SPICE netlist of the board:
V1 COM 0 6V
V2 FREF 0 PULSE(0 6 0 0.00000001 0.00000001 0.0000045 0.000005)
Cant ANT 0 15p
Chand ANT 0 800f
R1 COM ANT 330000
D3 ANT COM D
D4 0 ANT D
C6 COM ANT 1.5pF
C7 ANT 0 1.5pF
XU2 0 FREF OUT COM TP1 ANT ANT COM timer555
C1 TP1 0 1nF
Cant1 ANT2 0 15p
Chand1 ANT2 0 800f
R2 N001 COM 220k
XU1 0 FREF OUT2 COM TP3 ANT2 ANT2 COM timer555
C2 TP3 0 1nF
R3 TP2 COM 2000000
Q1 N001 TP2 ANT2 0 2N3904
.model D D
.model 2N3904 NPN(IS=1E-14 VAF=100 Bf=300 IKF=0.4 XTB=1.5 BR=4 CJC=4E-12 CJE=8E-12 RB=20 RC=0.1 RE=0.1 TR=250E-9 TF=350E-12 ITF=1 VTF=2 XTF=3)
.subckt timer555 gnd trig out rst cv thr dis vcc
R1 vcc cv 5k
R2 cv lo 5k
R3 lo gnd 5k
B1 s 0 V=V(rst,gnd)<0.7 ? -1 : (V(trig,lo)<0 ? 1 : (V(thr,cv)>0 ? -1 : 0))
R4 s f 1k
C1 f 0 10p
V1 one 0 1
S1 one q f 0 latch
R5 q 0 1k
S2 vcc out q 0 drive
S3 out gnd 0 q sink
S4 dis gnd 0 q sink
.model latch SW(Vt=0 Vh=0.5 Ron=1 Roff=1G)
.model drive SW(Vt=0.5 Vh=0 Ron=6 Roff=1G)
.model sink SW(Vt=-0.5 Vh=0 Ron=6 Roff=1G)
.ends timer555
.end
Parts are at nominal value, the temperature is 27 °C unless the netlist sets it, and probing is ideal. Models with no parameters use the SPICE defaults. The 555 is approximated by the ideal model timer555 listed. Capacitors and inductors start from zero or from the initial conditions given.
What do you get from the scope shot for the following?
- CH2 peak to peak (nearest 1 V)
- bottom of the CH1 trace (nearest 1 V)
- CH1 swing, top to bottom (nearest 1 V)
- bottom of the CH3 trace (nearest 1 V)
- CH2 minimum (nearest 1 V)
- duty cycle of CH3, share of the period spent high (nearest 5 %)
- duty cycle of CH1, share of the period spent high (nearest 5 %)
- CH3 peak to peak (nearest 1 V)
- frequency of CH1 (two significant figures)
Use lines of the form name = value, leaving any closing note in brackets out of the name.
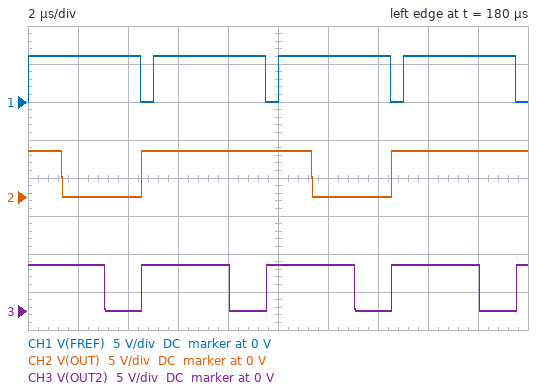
CH2 peak to peak = 6 V
bottom of the CH1 trace = 0 V
CH1 swing, top to bottom = 6 V
bottom of the CH3 trace = 0 V
CH2 minimum = 0 V
duty cycle of CH3, share of the period spent high = 70 %
duty cycle of CH1, share of the period spent high = 90 %
CH3 peak to peak = 6 V
frequency of CH1 = 200 kHz
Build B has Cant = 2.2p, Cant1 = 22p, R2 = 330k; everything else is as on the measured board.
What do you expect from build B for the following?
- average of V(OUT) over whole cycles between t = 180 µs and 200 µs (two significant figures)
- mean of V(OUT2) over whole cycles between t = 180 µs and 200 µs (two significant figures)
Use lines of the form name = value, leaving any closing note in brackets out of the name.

average of V(OUT) over whole cycles between t = 180 µs and 200 µs = 2.6 V
mean of V(OUT2) over whole cycles between t = 180 µs and 200 µs = 4.4 V
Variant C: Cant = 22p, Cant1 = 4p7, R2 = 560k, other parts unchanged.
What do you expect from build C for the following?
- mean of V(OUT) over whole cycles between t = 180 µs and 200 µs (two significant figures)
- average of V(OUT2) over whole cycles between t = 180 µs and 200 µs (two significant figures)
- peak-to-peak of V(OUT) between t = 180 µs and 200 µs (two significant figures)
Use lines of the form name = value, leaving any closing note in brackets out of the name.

mean of V(OUT) over whole cycles between t = 180 µs and 200 µs = 5.6 V
average of V(OUT2) over whole cycles between t = 180 µs and 200 µs = 3.3 V
peak-to-peak of V(OUT) between t = 180 µs and 200 µs = 6.0 V
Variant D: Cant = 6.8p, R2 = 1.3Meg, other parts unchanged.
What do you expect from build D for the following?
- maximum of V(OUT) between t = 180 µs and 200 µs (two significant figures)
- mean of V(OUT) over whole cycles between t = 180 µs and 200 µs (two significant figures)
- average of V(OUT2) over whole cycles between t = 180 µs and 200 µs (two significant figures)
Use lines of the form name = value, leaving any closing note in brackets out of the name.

maximum of V(OUT) between t = 180 µs and 200 µs = 6.0 V
mean of V(OUT) over whole cycles between t = 180 µs and 200 µs = 4.6 V
average of V(OUT2) over whole cycles between t = 180 µs and 200 µs = 5.9 V
